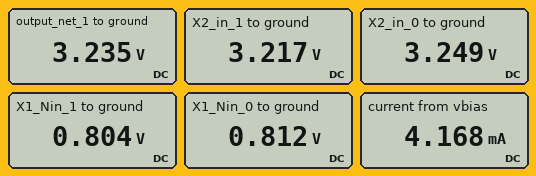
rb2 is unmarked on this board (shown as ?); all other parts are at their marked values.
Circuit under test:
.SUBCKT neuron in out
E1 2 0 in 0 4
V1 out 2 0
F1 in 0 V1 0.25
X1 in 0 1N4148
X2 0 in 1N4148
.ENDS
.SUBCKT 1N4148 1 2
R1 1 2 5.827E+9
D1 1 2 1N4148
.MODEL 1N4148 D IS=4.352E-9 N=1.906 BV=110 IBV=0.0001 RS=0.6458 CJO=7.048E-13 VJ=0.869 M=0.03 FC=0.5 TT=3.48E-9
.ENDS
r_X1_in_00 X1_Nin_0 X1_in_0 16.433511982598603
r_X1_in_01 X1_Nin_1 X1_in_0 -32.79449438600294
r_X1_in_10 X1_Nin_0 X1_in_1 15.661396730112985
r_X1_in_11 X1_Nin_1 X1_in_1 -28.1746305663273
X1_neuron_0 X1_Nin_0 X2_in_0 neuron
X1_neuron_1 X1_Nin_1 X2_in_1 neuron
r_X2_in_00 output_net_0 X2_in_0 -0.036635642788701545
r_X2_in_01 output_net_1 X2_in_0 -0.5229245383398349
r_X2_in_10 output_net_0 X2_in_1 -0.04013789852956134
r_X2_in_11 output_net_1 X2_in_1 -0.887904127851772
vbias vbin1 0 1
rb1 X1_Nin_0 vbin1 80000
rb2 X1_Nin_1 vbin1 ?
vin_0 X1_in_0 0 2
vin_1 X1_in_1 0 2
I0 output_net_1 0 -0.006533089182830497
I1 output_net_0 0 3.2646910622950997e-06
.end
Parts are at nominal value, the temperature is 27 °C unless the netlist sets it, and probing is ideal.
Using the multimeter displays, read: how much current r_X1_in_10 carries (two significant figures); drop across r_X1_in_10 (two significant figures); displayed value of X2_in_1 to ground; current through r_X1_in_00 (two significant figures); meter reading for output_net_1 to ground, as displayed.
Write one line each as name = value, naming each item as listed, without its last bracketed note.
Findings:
how much current r_X1_in_10 carries = 76 mA
drop across r_X1_in_10 = 1.2 V
displayed value of X2_in_1 to ground = 3.217 V
current through r_X1_in_00 = 72 mA
meter reading for output_net_1 to ground, as displayed = 3.235 V
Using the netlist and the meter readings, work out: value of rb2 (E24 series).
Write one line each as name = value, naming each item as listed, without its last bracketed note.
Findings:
value of rb2 = 47 Ω
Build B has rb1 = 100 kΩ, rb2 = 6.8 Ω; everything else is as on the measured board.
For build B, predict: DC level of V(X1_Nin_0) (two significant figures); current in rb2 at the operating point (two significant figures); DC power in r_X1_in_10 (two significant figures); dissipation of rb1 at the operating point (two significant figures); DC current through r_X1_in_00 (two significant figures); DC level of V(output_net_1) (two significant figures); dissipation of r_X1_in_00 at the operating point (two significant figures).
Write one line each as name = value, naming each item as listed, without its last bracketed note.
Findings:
DC level of V(X1_Nin_0) = 830 mV
current in rb2 at the operating point = 26 mA
DC power in r_X1_in_10 = 87 mW
dissipation of rb1 at the operating point = 290 nW
DC current through r_X1_in_00 = 71 mA
DC level of V(output_net_1) = 3.3 V
dissipation of r_X1_in_00 at the operating point = 83 mW
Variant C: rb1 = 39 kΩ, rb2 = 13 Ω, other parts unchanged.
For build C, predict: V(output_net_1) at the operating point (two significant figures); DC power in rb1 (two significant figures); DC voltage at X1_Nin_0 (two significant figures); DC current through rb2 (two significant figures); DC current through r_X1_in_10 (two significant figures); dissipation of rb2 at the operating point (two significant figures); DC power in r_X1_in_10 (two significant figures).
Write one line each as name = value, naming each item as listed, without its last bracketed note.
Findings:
V(output_net_1) at the operating point = 3.3 V
DC power in rb1 = 820 nW
DC voltage at X1_Nin_0 = 820 mV
DC current through rb2 = 14 mA
DC current through r_X1_in_10 = 75 mA
dissipation of rb2 at the operating point = 2.7 mW
DC power in r_X1_in_10 = 89 mW
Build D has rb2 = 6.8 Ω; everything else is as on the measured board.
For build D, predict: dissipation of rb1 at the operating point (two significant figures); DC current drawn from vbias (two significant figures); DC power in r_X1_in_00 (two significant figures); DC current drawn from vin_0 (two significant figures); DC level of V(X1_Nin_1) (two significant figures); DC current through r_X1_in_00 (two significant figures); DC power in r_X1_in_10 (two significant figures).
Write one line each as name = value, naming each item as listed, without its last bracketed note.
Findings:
dissipation of rb1 at the operating point = 360 nW
DC current drawn from vbias = 26 mA
DC power in r_X1_in_00 = 83 mW
DC current drawn from vin_0 = 35 mA
DC level of V(X1_Nin_1) = 820 mV
DC current through r_X1_in_00 = 71 mA
DC power in r_X1_in_10 = 87 mW
